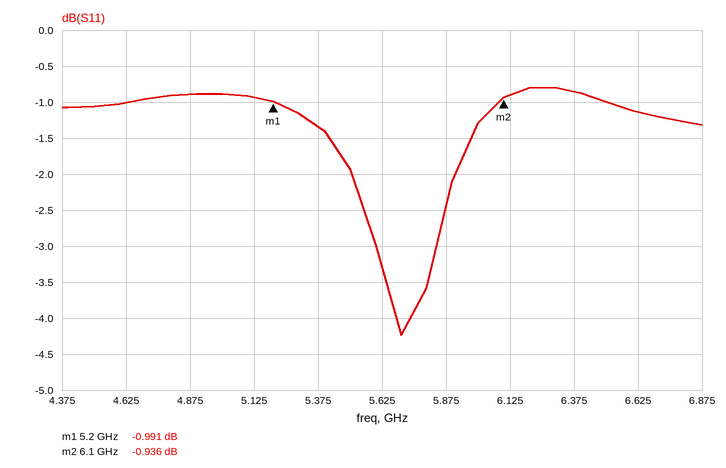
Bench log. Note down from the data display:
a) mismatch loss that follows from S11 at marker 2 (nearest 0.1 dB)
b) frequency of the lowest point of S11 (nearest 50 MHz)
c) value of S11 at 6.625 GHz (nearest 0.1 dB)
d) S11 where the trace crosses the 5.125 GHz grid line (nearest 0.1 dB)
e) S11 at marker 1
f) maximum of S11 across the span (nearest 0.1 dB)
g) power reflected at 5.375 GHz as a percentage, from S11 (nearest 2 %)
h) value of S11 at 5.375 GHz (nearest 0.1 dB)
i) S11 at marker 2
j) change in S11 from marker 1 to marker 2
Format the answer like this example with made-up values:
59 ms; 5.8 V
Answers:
7.1 dB; 5.70 GHz; -1.1 dB; -0.9 dB; -0.991 dB; -0.8 dB; 74 %; -1.3 dB; -0.936 dB; 0.055 dB
